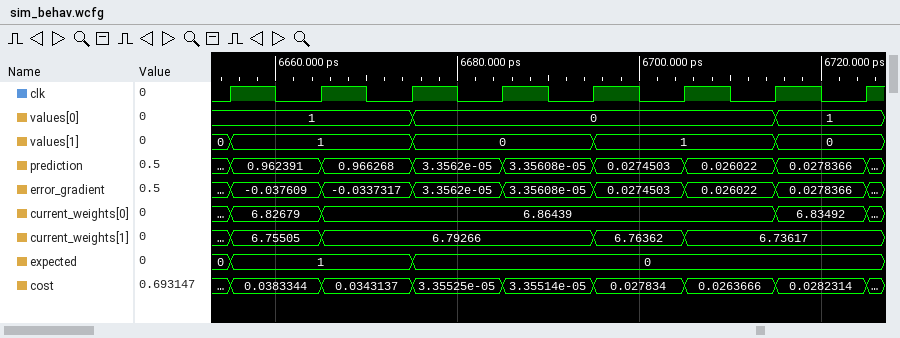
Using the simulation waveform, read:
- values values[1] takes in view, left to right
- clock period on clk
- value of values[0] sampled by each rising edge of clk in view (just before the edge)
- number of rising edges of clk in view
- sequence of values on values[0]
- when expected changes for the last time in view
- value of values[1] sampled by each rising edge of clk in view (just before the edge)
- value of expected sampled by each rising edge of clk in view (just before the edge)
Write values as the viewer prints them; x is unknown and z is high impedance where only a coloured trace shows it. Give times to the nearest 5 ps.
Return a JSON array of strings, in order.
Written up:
["0, 1, 0, 1, 0", "10 ps", "1, 1, 1, 0, 0, 0, 0, 1", "8", "1, 0, 1", "6675 ps", "0, 1, 1, 0, 0, 1, 1, 0", "0, 1, 1, 0, 0, 0, 0, 0"]
